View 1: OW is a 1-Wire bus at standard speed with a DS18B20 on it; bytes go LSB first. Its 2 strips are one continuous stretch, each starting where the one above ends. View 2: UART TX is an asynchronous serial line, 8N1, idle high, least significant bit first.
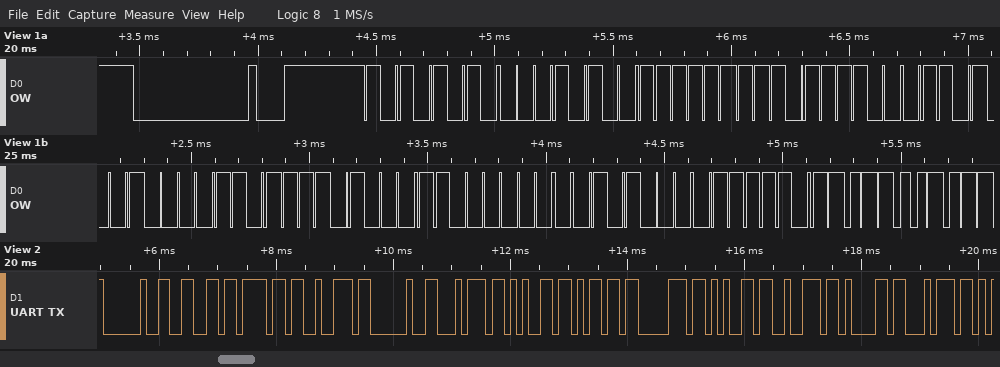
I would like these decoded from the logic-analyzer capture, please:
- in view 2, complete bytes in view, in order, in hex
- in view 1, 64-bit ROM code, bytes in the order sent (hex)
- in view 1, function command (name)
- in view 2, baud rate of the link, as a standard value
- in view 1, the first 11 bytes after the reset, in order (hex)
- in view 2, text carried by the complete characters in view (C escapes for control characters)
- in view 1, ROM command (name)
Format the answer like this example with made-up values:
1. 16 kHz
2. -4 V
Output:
1. 0x20 0x66 0x6F 0x72 0x20 0x74 0x65 0x6D 0x70 0x65 0x72 0x61 0x74
2. 28 FF 3D 96 B0 17 03 14
3. Read Scratchpad
4. 9600 baud
5. 55 28 FF 3D 96 B0 17 03 14 BE 4D
6. " for temperat"
7. Match ROM
